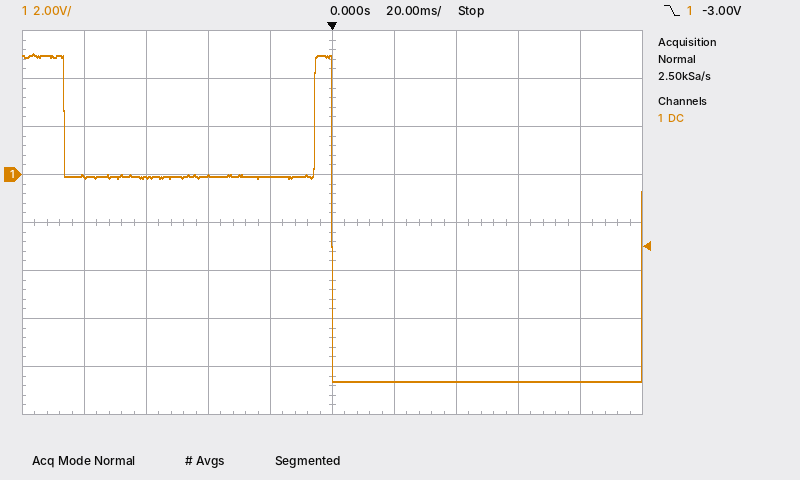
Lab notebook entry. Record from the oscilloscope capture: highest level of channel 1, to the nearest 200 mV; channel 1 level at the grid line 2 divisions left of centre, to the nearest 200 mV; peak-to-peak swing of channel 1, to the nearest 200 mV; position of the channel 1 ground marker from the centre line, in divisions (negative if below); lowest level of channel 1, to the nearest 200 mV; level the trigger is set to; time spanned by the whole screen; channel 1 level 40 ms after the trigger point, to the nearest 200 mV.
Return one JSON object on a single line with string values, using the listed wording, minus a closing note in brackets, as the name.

{"highest level of channel 1, to the nearest 200 mV": "5.0 V", "channel 1 level at the grid line 2 divisions left of centre, to the nearest 200 mV": "0.0 V", "peak-to-peak swing of channel 1, to the nearest 200 mV": "13.6 V", "position of the channel 1 ground marker from the centre line, in divisions": "+1.0 div", "lowest level of channel 1, to the nearest 200 mV": "-8.6 V", "level the trigger is set to": "-3.00 V", "time spanned by the whole screen": "200 ms", "channel 1 level 40 ms after the trigger point, to the nearest 200 mV": "-8.6 V"}
